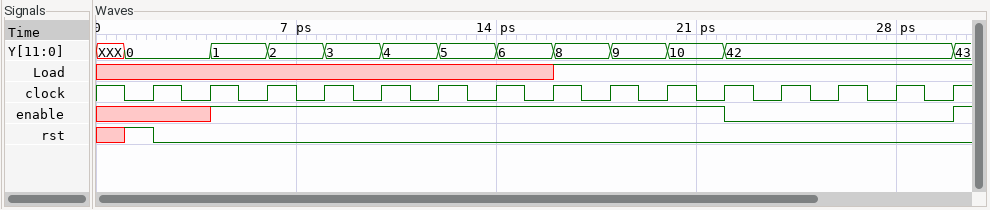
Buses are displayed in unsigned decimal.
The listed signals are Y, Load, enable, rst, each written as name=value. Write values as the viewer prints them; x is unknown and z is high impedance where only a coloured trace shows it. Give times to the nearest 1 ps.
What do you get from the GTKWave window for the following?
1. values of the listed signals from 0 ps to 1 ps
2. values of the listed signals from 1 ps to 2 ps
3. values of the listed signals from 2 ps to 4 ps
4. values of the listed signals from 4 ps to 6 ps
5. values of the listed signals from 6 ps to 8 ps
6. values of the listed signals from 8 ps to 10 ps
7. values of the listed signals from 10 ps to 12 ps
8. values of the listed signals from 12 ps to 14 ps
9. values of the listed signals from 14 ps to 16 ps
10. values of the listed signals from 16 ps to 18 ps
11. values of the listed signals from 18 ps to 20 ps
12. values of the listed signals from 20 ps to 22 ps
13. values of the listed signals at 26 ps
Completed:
Y=XXX, Load=x, enable=x, rst=x
Y=0, Load=x, enable=x, rst=1
Y=0, Load=x, enable=x, rst=0
Y=1, Load=x, enable=1, rst=0
Y=2, Load=x, enable=1, rst=0
Y=3, Load=x, enable=1, rst=0
Y=4, Load=x, enable=1, rst=0
Y=5, Load=x, enable=1, rst=0
Y=6, Load=x, enable=1, rst=0
Y=8, Load=1, enable=1, rst=0
Y=9, Load=1, enable=1, rst=0
Y=10, Load=1, enable=1, rst=0
Y=42, Load=1, enable=0, rst=0
